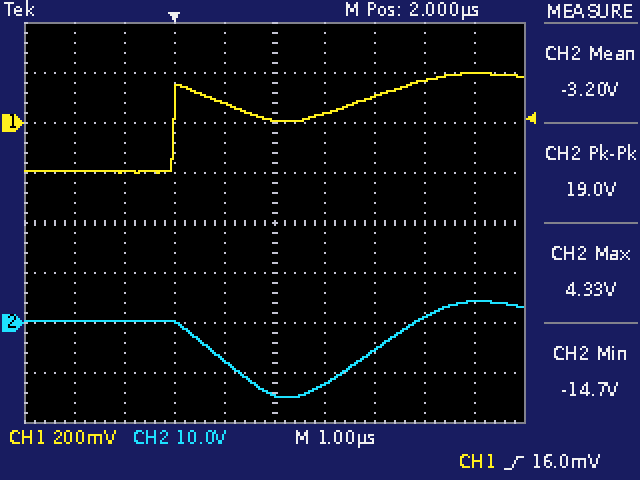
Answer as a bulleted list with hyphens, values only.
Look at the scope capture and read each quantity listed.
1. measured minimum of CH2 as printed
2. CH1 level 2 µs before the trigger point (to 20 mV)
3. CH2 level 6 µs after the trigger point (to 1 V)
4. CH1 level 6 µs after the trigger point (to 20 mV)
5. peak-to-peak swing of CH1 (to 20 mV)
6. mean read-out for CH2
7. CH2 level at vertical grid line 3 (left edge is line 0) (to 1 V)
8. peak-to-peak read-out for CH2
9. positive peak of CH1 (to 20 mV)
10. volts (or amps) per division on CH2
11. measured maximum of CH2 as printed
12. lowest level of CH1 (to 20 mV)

- -14.7 V
- -200 mV
- 4 V
- 200 mV
- 400 mV
- -3.20 V
- 0 V
- 19.0 V
- 200 mV
- 10 V
- 4.33 V
- -200 mV
